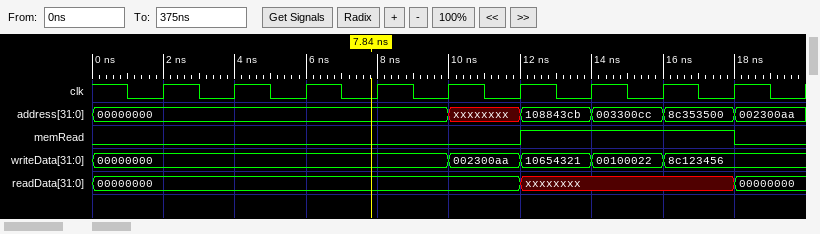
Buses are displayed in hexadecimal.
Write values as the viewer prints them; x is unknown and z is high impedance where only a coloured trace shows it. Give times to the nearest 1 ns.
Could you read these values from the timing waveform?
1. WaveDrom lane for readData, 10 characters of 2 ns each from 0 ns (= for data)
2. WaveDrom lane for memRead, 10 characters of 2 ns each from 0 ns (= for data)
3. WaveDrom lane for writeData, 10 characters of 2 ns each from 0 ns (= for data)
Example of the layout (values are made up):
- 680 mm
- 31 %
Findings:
- {name: 'readData', wave: '=.....x..=', data: '00000000 00000000'}
- {name: 'memRead', wave: '0.....1..0'}
- {name: 'writeData', wave: '=....====.', data: '00000000 002300aa 10654321 00100022 8c123456'}
